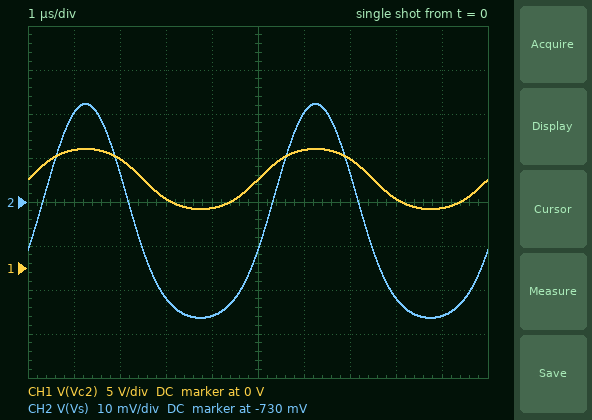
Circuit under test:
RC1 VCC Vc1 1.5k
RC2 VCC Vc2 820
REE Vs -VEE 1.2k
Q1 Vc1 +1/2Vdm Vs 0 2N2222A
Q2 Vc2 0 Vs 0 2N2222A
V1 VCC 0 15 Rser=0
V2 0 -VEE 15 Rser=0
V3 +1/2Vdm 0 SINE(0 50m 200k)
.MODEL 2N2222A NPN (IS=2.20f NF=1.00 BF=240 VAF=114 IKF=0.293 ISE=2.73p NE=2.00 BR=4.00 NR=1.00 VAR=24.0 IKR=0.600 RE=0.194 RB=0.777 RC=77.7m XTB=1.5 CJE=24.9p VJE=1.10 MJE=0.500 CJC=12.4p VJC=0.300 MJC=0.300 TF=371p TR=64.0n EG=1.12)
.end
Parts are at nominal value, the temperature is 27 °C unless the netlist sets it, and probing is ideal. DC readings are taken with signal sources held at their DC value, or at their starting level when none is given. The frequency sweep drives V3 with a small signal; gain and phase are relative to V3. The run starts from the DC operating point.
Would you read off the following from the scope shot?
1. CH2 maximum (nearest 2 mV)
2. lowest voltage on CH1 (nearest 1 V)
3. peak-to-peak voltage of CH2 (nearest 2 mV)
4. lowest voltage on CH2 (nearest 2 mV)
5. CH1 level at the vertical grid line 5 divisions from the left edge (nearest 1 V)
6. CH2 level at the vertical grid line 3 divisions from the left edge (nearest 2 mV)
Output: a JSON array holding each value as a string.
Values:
["-708 mV", "7 V", "48 mV", "-756 mV", "10 V", "-752 mV"]
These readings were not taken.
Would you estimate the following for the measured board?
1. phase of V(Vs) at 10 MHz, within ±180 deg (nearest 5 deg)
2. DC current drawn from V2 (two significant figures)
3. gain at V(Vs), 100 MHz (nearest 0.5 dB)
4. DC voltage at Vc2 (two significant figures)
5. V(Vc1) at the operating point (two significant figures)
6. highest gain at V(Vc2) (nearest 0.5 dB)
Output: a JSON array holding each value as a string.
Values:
["0 deg", "12 mA", "-6.0 dB", "10 V", "6.3 V", "38.5 dB"]
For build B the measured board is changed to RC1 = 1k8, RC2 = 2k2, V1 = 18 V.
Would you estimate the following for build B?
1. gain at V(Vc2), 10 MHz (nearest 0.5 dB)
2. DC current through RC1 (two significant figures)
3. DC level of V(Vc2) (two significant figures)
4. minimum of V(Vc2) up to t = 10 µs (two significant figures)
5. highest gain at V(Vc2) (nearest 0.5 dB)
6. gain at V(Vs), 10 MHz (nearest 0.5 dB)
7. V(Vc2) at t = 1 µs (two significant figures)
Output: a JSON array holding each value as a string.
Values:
["44.5 dB", "6.0 mA", "5.1 V", "-730 mV", "46.5 dB", "-6.0 dB", "14 V"]
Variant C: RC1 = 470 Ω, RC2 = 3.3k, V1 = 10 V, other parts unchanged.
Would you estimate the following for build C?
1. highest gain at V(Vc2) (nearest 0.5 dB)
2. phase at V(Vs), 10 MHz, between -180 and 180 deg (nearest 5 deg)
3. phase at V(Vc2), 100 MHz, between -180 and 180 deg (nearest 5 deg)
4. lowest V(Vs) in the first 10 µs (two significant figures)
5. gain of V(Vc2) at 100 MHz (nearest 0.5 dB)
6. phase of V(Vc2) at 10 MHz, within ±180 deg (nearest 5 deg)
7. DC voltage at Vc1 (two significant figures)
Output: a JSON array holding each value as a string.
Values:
["3.0 dB", "-5 deg", "0 deg", "-780 mV", "-21.0 dB", "-60 deg", "6.4 V"]
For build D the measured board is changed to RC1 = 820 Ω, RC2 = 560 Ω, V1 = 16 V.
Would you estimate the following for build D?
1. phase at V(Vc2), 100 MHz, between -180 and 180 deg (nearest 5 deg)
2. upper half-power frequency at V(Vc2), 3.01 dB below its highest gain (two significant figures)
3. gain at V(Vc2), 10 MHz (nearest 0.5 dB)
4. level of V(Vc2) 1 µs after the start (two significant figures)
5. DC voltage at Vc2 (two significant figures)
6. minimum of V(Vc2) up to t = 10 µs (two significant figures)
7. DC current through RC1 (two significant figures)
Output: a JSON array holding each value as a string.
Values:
["-60 deg", "61 MHz", "35.0 dB", "15 V", "13 V", "10 V", "5.9 mA"]
